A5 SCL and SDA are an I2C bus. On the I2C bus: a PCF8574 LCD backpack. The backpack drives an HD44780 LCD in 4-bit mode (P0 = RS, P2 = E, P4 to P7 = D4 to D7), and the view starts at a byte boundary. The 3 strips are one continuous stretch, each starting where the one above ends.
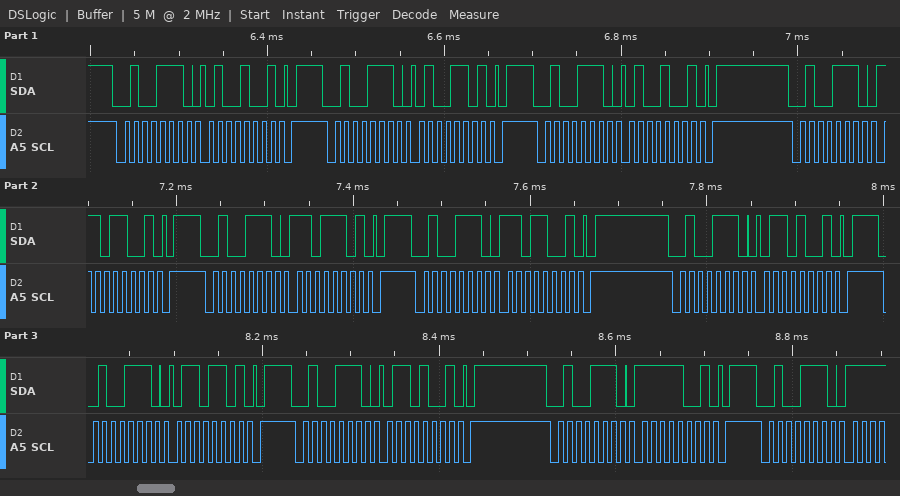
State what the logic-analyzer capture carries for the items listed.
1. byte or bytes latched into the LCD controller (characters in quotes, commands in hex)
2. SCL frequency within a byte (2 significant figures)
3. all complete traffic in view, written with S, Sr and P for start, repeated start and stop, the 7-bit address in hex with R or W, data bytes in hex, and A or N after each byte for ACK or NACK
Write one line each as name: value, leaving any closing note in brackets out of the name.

byte or bytes latched into the LCD controller: 'M'
SCL frequency within a byte: 100 kHz
all complete traffic in view, written with S, Sr and P for start, repeated start and stop, the 7-bit address in hex with R or W, data bytes in hex, and A or N after each byte for ACK or NACK: S 27W A 49 A P S 27W A 4D A P S 27W A 49 A P S 27W A D9 A P S 27W A DD A P S 27W A D9 A P S 27W A 69 A P S 27W A 6D A P S 27W A 69 A P S 27W A F9 A P S 27W A
